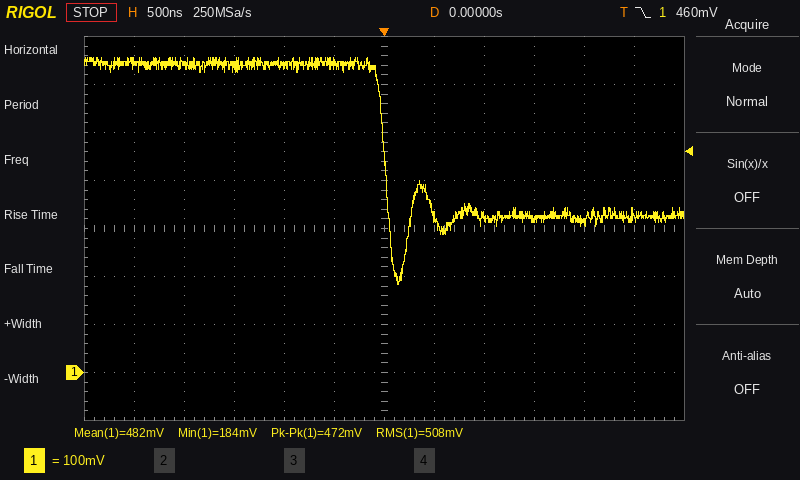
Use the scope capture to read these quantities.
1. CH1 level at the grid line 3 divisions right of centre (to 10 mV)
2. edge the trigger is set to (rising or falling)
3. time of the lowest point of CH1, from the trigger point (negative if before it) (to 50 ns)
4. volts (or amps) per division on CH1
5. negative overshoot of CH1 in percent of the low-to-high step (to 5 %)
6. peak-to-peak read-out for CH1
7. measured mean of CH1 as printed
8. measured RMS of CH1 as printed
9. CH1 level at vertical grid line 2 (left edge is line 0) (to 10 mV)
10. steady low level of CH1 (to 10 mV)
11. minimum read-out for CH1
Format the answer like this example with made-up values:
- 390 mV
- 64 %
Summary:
- 320 mV
- falling
- +150 ns
- 100 mV
- 45 %
- 472 mV
- 482 mV
- 508 mV
- 640 mV
- 320 mV
- 184 mV
